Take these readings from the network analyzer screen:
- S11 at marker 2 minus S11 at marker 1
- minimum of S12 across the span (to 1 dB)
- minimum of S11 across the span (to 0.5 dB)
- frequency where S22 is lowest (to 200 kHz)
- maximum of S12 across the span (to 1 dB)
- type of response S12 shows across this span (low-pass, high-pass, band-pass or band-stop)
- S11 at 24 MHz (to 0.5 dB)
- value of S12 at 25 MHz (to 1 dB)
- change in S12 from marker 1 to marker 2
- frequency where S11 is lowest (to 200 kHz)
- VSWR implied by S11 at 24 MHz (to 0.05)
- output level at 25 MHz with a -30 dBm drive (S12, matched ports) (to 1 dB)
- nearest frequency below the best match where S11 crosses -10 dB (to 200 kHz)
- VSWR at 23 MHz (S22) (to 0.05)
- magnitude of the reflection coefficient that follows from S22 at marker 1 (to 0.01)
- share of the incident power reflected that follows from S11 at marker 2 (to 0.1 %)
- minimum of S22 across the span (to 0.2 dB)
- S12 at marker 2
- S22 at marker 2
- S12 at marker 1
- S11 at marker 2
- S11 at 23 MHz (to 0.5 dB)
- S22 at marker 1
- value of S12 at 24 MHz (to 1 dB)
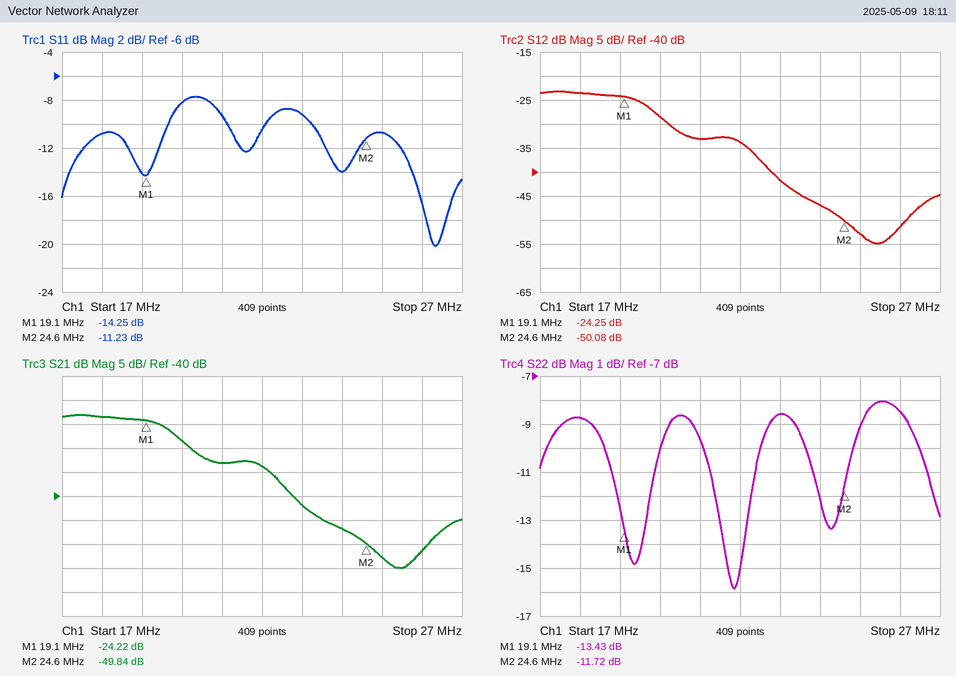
3.02 dB
-55 dB
-20.0 dB
21.8 MHz
-23 dB
low-pass
-14.0 dB
-53 dB
-25.83 dB
26.4 MHz
1.50
-83 dBm
23.2 MHz
2.20
0.21
7.5 %
-15.8 dB
-50.08 dB
-11.72 dB
-24.25 dB
-11.23 dB
-9.0 dB
-13.43 dB
-47 dB
